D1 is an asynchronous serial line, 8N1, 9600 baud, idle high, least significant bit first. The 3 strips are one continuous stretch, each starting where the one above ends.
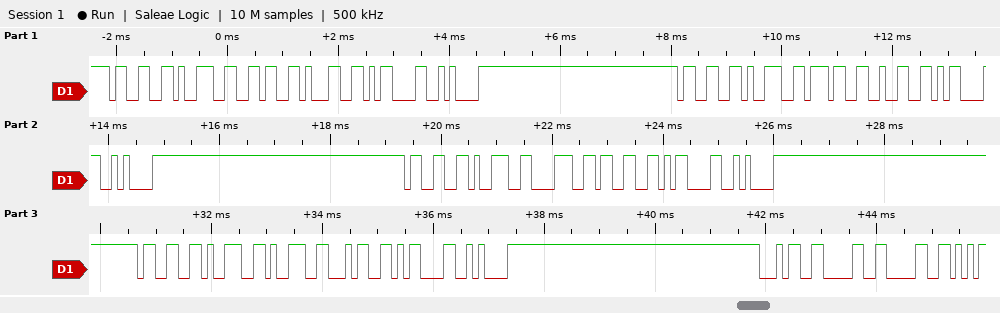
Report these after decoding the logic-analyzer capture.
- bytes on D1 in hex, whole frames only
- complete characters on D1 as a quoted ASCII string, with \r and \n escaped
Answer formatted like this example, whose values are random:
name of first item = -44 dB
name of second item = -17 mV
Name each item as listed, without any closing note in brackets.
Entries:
bytes on D1 in hex, whole frames only = 33 39 36 31 0D 0A 33 39 37 32 0D 0A 33 39 38 33 0D 0A 33 39 39 34 0D 0A 34 30 30
complete characters on D1 as a quoted ASCII string, with \r and \n escaped = "3961\r\n3972\r\n3983\r\n3994\r\n400"
